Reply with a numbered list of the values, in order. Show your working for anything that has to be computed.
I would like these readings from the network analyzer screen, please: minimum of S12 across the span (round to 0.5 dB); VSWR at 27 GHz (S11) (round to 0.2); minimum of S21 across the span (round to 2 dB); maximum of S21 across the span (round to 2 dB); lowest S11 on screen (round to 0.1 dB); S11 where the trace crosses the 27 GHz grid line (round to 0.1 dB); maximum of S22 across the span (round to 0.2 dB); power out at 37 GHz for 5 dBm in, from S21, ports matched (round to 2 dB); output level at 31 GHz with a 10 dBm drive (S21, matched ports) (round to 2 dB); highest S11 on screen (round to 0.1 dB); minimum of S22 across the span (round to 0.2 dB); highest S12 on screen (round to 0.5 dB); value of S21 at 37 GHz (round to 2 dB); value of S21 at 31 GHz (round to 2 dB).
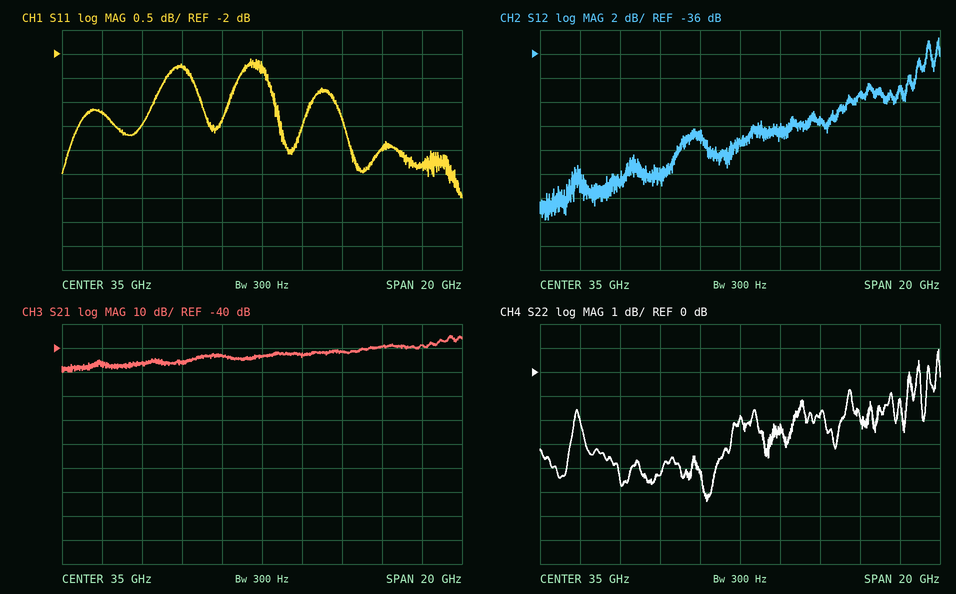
1. -50.0 dB
2. |Γ| = 10^(-3.2/20) = 0.6918; VSWR = (1 + 0.6918)/(1 − 0.6918) ≈ 5.49, so 5.4 to the nearest 0.2
3. -50 dB
4. -34 dB
5. -5.0 dB
6. -3.2 dB
7. 1.0 dB
8. 5 dBm + (-42 dB) = -38 dBm
9. 10 dBm + (-46 dB) = -36 dBm
10. -2.1 dB
11. -5.4 dB
12. -34.5 dB
13. -42 dB
14. -46 dB
